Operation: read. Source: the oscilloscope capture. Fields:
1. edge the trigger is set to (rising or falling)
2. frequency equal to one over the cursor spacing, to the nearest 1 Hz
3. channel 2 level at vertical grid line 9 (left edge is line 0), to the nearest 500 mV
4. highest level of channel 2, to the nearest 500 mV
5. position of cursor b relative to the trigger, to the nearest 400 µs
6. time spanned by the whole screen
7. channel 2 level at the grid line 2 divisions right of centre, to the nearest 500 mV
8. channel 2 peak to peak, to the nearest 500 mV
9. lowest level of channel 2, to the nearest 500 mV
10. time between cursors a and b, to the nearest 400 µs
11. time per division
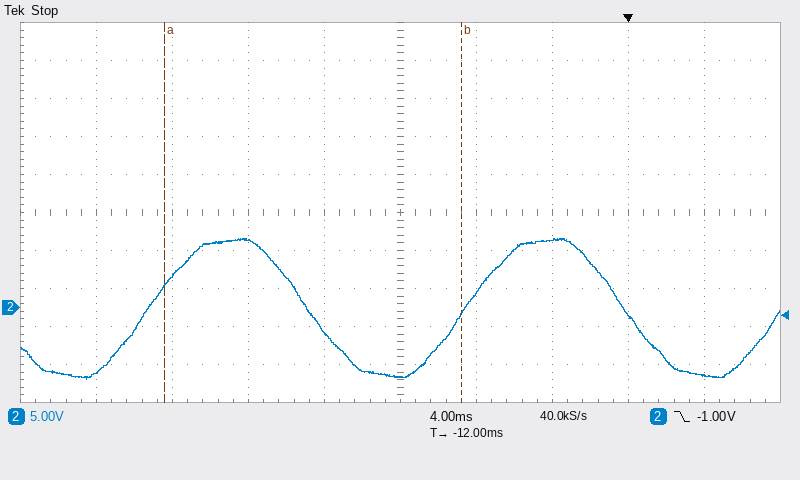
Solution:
falling
64 Hz
-9.0 V
9.0 V
-8.8 ms
40 ms
9.0 V
18.5 V
-9.5 V
15.6 ms
4 ms
